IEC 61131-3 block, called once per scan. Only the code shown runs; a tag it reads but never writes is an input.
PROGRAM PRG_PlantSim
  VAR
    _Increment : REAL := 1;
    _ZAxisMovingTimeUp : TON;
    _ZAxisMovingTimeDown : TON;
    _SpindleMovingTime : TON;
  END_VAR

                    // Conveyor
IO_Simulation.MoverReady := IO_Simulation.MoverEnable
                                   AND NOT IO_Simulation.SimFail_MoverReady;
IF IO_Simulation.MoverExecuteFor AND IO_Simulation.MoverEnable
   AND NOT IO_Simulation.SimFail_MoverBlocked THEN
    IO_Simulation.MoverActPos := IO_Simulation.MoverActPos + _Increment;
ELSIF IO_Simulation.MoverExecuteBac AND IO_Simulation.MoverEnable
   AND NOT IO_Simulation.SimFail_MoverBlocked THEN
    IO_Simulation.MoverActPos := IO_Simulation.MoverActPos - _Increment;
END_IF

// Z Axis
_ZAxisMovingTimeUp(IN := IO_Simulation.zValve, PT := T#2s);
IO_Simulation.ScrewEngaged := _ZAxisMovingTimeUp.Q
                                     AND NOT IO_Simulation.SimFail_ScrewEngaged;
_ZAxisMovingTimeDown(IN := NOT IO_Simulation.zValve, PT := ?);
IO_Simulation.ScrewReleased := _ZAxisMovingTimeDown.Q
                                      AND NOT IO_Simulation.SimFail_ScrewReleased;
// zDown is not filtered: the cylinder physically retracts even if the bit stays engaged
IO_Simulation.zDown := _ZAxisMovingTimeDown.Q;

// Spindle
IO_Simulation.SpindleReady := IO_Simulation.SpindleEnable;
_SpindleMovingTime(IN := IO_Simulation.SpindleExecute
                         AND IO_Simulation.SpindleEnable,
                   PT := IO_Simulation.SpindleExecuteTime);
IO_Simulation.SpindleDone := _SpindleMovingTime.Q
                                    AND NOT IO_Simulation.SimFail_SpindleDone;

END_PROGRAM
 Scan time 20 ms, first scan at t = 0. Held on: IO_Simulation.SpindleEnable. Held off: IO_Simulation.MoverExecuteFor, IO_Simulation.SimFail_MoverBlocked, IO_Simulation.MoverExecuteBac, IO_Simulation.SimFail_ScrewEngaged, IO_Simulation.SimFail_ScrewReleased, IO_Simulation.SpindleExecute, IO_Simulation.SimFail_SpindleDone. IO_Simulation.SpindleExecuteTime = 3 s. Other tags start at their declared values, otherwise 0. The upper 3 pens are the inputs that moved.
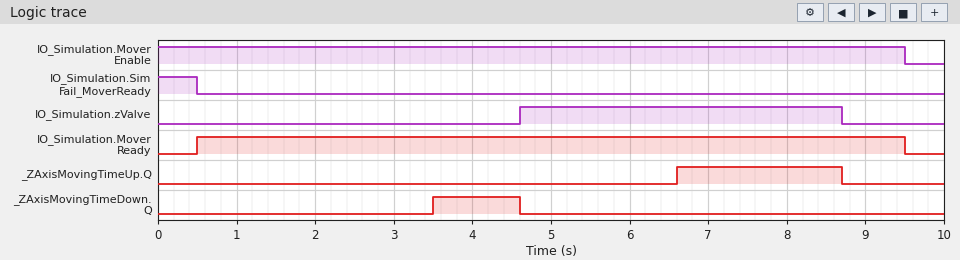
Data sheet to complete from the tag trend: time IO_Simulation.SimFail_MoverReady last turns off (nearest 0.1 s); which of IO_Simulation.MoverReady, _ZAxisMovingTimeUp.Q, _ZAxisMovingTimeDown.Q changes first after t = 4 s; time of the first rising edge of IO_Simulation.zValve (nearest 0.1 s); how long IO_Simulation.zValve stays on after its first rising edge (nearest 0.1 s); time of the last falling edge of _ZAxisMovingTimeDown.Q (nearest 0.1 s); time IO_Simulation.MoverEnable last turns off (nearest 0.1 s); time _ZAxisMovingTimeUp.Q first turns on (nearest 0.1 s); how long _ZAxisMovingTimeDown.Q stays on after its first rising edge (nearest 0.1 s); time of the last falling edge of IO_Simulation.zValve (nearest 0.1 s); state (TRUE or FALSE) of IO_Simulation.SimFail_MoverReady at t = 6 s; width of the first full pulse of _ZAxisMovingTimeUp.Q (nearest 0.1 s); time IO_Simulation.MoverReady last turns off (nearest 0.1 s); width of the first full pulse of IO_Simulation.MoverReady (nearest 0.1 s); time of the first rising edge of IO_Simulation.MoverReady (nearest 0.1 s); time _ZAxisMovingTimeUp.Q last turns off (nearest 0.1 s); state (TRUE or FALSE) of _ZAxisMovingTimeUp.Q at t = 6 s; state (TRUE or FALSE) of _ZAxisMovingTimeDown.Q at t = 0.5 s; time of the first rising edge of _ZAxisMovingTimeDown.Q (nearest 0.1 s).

0.5 s
_ZAxisMovingTimeDown.Q
4.6 s
4.1 s
4.6 s
9.5 s
6.6 s
1.1 s
8.7 s
FALSE
2.1 s
9.5 s
9.0 s
0.5 s
8.7 s
FALSE
FALSE
3.5 s
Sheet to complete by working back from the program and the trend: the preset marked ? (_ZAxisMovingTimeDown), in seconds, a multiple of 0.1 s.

3.5 s
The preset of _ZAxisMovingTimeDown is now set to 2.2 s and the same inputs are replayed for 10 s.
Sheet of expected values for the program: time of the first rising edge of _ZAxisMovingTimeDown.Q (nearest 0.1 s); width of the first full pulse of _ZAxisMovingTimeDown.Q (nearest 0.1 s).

2.2 s
2.4 s
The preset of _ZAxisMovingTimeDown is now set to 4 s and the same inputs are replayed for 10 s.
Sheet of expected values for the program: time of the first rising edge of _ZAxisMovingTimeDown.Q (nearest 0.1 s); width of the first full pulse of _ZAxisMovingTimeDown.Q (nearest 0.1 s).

4.0 s
0.6 s
